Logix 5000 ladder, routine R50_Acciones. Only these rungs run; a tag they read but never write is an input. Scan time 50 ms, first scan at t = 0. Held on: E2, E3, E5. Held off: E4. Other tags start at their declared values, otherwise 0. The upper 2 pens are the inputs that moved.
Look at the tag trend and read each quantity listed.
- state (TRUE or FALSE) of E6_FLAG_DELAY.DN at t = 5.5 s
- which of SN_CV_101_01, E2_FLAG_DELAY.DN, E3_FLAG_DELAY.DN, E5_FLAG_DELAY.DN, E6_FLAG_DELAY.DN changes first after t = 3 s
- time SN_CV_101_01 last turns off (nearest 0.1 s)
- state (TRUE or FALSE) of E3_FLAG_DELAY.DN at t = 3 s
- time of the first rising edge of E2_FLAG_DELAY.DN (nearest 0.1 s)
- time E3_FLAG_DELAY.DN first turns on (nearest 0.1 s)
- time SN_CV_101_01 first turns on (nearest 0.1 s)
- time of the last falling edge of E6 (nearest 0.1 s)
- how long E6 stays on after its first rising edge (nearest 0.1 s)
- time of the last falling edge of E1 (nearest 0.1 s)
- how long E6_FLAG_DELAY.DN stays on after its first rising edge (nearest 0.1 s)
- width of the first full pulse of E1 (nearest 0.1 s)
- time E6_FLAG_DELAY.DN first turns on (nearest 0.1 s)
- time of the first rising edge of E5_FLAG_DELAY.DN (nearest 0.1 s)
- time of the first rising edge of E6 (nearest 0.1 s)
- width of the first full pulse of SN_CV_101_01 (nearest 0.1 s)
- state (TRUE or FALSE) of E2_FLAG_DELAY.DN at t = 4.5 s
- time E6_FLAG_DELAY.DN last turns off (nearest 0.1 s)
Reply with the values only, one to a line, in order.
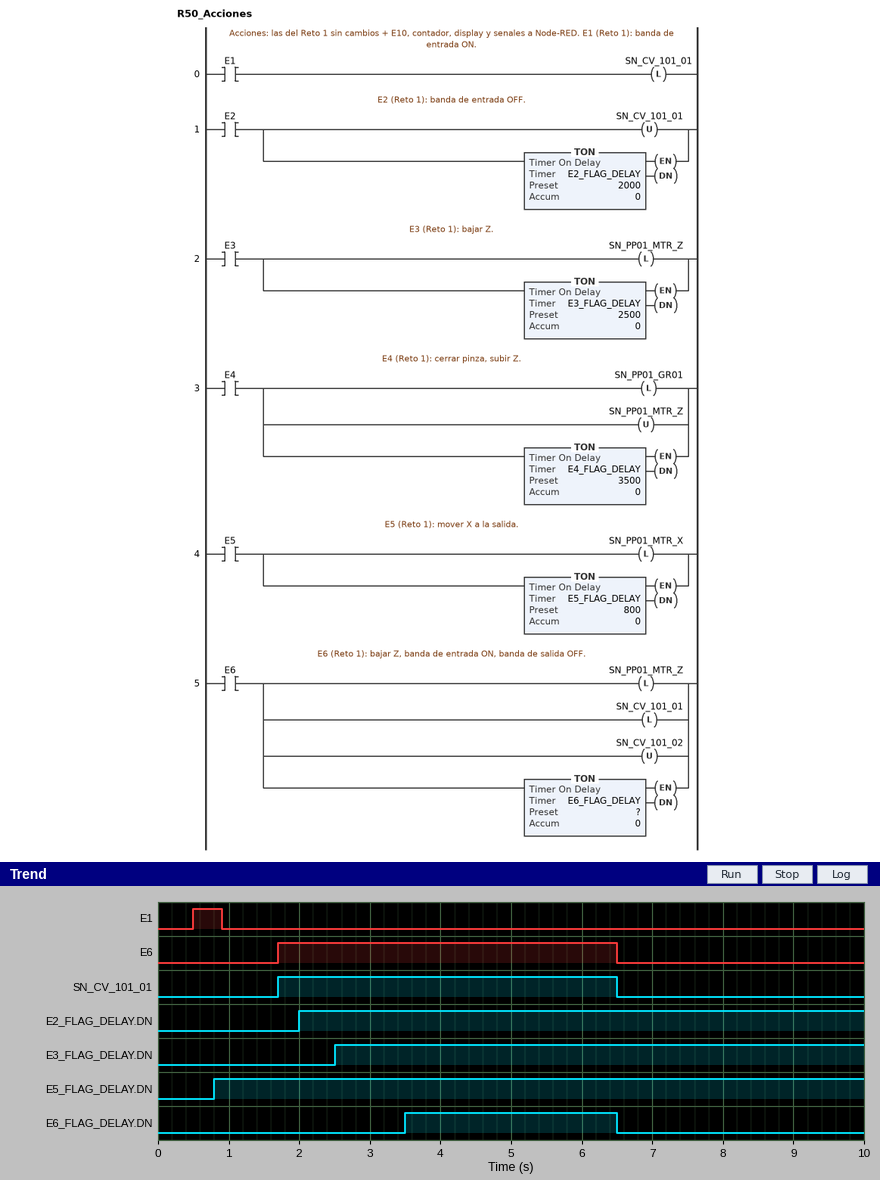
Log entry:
TRUE
E6_FLAG_DELAY.DN
6.5 s
TRUE
2.0 s
2.5 s
1.7 s
6.5 s
4.8 s
0.9 s
3.0 s
0.4 s
3.5 s
0.8 s
1.7 s
4.8 s
TRUE
6.5 s
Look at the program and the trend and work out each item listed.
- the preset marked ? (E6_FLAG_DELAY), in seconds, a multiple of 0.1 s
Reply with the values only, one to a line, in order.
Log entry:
1.8 s
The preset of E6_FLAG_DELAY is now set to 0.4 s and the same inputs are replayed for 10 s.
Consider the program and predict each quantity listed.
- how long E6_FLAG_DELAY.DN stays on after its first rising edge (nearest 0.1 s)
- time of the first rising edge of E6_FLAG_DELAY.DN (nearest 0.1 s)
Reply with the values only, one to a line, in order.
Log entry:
4.4 s
2.1 s
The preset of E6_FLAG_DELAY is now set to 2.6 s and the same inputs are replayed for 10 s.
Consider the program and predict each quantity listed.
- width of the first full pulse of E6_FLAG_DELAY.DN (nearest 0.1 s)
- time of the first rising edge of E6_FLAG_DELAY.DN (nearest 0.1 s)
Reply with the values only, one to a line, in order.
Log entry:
2.2 s
4.3 s
